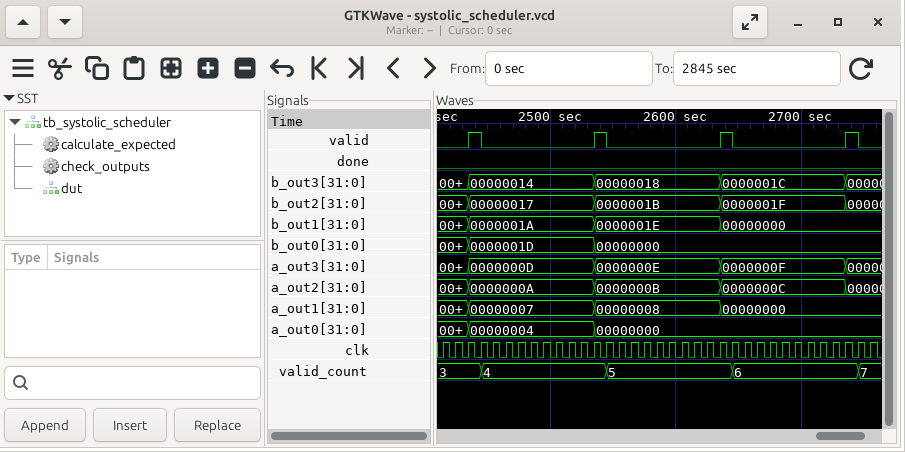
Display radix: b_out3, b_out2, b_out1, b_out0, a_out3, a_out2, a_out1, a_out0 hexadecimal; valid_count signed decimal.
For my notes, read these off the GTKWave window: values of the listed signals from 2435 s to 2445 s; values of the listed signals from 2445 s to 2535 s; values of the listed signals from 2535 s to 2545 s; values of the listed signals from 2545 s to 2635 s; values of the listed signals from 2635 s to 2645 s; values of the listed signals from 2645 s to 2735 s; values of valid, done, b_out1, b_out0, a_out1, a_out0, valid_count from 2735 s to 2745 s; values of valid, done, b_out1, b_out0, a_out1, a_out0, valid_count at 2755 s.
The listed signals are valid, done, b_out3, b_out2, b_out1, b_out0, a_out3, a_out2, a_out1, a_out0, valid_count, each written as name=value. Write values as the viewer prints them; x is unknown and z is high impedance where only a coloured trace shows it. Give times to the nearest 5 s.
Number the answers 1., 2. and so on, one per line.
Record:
1. valid=1, done=0, b_out3=00000014, b_out2=00000017, b_out1=0000001A, b_out0=0000001D, a_out3=0000000D, a_out2=0000000A, a_out1=00000007, a_out0=00000004, valid_count=3
2. valid=0, done=0, b_out3=00000014, b_out2=00000017, b_out1=0000001A, b_out0=0000001D, a_out3=0000000D, a_out2=0000000A, a_out1=00000007, a_out0=00000004, valid_count=4
3. valid=1, done=0, b_out3=00000018, b_out2=0000001B, b_out1=0000001E, b_out0=00000000, a_out3=0000000E, a_out2=0000000B, a_out1=00000008, a_out0=00000000, valid_count=4
4. valid=0, done=0, b_out3=00000018, b_out2=0000001B, b_out1=0000001E, b_out0=00000000, a_out3=0000000E, a_out2=0000000B, a_out1=00000008, a_out0=00000000, valid_count=5
5. valid=1, done=0, b_out3=0000001C, b_out2=0000001F, b_out1=00000000, b_out0=00000000, a_out3=0000000F, a_out2=0000000C, a_out1=00000000, a_out0=00000000, valid_count=5
6. valid=0, done=0, b_out3=0000001C, b_out2=0000001F, b_out1=00000000, b_out0=00000000, a_out3=0000000F, a_out2=0000000C, a_out1=00000000, a_out0=00000000, valid_count=6
7. valid=1, done=0, b_out1=00000000, b_out0=00000000, a_out1=00000000, a_out0=00000000, valid_count=6
8. valid=0, done=0, b_out1=00000000, b_out0=00000000, a_out1=00000000, a_out0=00000000, valid_count=7
